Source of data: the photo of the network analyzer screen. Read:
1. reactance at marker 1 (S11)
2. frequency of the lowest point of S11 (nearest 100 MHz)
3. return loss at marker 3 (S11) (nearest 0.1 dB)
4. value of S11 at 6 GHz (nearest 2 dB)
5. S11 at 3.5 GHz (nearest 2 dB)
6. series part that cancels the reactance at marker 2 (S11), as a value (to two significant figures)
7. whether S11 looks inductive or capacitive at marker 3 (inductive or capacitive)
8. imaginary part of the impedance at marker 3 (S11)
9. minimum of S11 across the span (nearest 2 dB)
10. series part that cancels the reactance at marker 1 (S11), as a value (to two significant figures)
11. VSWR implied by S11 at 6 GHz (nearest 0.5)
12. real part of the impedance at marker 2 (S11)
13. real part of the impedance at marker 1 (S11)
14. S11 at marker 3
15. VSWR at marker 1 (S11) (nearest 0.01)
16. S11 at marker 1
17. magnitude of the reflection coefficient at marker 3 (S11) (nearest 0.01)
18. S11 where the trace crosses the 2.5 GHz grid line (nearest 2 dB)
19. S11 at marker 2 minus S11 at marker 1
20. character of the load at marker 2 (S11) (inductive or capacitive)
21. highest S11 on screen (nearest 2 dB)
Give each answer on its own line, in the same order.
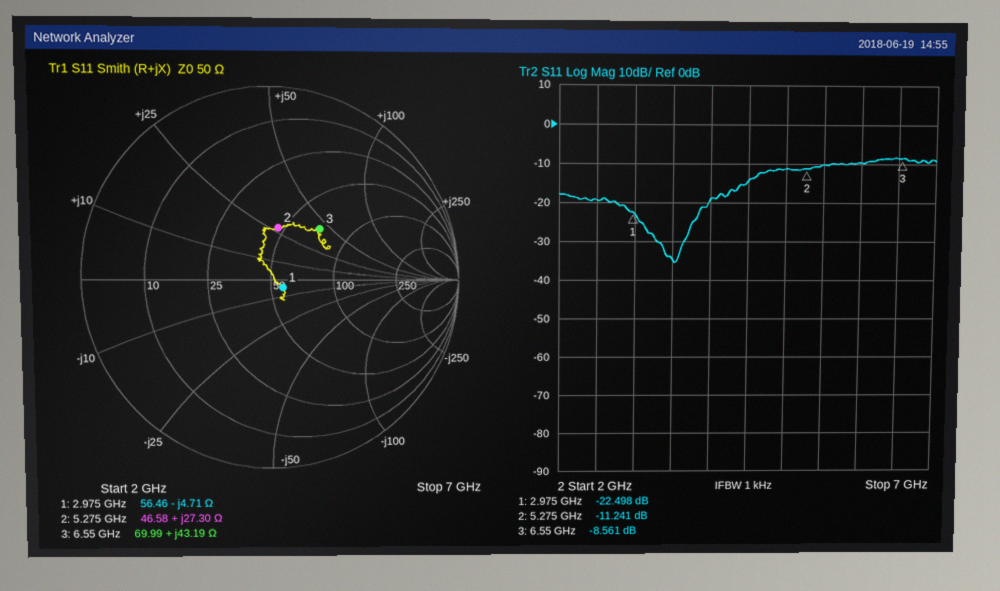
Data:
-4.71 Ω
3.5 GHz
8.6 dB
-10 dB
-34 dB
1.1 pF
inductive
+43.19 Ω
-36 dB
250 pH
2.0
46.58 Ω
56.46 Ω
-8.561 dB
1.16
-22.498 dB
0.37
-20 dB
11.257 dB
inductive
-8 dB
